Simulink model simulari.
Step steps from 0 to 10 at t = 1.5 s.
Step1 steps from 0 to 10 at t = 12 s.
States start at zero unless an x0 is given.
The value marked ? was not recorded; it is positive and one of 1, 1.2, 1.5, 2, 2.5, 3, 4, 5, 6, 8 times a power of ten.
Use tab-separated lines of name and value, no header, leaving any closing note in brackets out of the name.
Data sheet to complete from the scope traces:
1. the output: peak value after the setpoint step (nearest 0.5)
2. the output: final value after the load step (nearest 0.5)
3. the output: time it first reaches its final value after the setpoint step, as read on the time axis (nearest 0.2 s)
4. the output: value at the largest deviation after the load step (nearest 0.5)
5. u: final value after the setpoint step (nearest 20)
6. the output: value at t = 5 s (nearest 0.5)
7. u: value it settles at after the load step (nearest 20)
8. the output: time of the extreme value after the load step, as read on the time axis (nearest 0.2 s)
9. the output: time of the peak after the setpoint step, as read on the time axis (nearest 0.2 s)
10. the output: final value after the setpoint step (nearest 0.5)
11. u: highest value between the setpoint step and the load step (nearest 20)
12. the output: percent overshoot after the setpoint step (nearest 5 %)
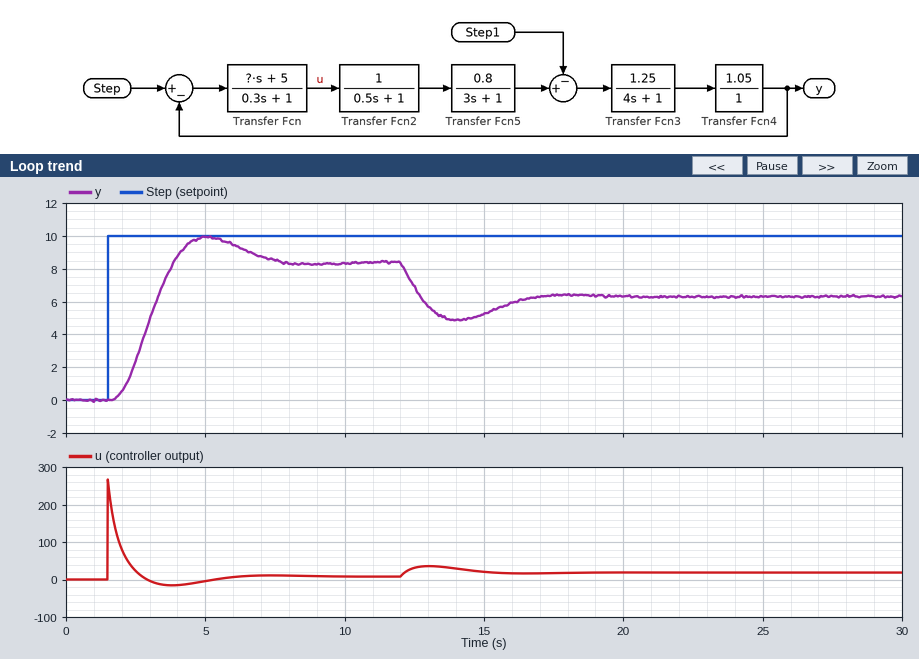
the output: peak value after the setpoint step	10.0
the output: final value after the load step	6.5
the output: time it first reaches its final value after the setpoint step, as read on the time axis	3.8 s
the output: value at the largest deviation after the load step	5.0
u: final value after the setpoint step	0
the output: value at t = 5 s	10.0
u: value it settles at after the load step	20
the output: time of the extreme value after the load step, as read on the time axis	14.0 s
the output: time of the peak after the setpoint step, as read on the time axis	5.0 s
the output: final value after the setpoint step	8.5
u: highest value between the setpoint step and the load step	260
the output: percent overshoot after the setpoint step	20 %
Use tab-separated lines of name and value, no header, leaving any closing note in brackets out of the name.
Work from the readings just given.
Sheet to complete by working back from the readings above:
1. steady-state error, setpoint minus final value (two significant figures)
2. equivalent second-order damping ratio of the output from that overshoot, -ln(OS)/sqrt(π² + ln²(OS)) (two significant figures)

steady-state error, setpoint minus final value	1.5
equivalent second-order damping ratio of the output from that overshoot, -ln(OS)/sqrt(π² + ln²(OS))	0.46
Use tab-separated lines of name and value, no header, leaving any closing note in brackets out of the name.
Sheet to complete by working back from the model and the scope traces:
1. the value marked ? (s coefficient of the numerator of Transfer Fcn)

the value marked ?	8
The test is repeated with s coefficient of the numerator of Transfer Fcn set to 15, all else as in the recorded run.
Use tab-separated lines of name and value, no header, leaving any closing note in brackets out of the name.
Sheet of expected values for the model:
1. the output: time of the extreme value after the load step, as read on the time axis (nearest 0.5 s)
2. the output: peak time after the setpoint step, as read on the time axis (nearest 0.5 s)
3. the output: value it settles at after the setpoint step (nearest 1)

the output: time of the extreme value after the load step, as read on the time axis	13.5 s
the output: peak time after the setpoint step, as read on the time axis	4.0 s
the output: value it settles at after the setpoint step	8
